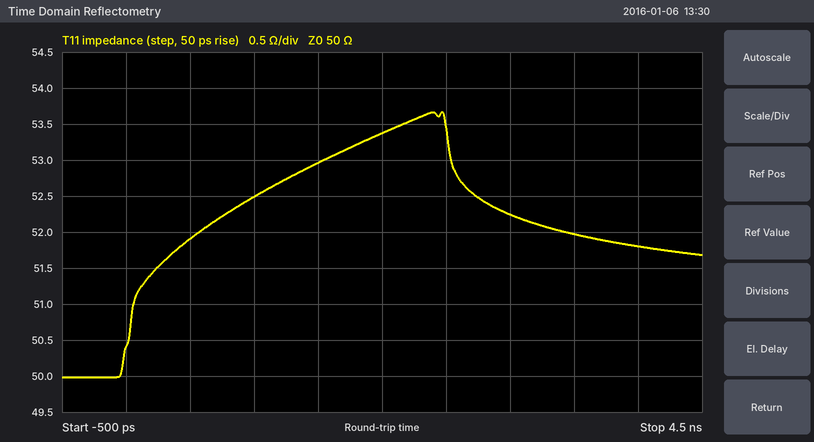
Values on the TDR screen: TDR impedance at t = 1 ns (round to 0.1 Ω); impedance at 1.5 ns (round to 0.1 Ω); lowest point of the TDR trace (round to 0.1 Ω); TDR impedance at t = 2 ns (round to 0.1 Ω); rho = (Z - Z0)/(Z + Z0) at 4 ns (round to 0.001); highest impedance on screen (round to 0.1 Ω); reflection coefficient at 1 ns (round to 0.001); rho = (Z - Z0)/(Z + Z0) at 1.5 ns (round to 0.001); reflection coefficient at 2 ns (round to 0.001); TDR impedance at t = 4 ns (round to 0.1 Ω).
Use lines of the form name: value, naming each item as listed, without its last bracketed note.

TDR impedance at t = 1 ns: 52.5 Ω
impedance at 1.5 ns: 53.0 Ω
lowest point of the TDR trace: 50.0 Ω
TDR impedance at t = 2 ns: 53.4 Ω
rho = (Z - Z0)/(Z + Z0) at 4 ns: +0.018
highest impedance on screen: 53.7 Ω
reflection coefficient at 1 ns: +0.024
rho = (Z - Z0)/(Z + Z0) at 1.5 ns: +0.029
reflection coefficient at 2 ns: +0.033
TDR impedance at t = 4 ns: 51.8 Ω
